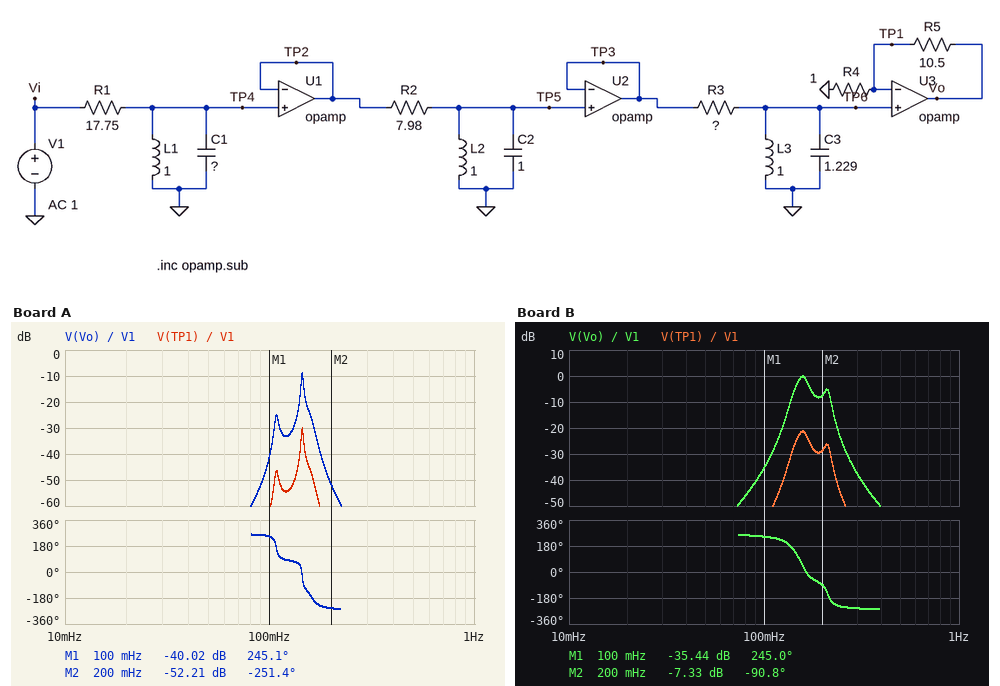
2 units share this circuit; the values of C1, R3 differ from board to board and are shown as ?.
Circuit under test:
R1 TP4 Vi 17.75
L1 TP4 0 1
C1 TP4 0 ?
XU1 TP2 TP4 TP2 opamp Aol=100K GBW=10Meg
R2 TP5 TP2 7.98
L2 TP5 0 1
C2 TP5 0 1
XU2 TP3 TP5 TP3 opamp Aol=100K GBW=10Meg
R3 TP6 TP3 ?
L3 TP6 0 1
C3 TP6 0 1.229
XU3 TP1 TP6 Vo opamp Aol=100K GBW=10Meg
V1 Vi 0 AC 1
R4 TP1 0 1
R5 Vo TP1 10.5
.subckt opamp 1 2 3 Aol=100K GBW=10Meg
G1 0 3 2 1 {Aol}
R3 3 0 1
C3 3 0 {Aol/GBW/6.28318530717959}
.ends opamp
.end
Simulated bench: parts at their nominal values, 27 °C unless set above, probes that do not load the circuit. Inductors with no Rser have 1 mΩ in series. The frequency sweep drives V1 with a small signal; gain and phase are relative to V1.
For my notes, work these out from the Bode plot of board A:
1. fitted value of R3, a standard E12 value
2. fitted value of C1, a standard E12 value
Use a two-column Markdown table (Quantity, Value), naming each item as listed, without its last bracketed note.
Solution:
| Quantity | Value |
|---|---|
| fitted value of R3, a standard E12 value | 47 Ω |
| fitted value of C1, a standard E12 value | 2.2 F |
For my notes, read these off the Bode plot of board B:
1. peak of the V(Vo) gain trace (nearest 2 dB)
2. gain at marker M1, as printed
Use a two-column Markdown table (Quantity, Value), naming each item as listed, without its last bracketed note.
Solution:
| Quantity | Value |
|---|---|
| peak of the V(Vo) gain trace | 0 dB |
| gain at marker M1, as printed | -35.44 dB |
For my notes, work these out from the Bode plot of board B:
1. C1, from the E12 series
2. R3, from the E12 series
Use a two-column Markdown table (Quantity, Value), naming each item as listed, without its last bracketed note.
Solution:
| Quantity | Value |
|---|---|
| C1, from the E12 series | 560 mF |
| R3, from the E12 series | 4.7 Ω |
